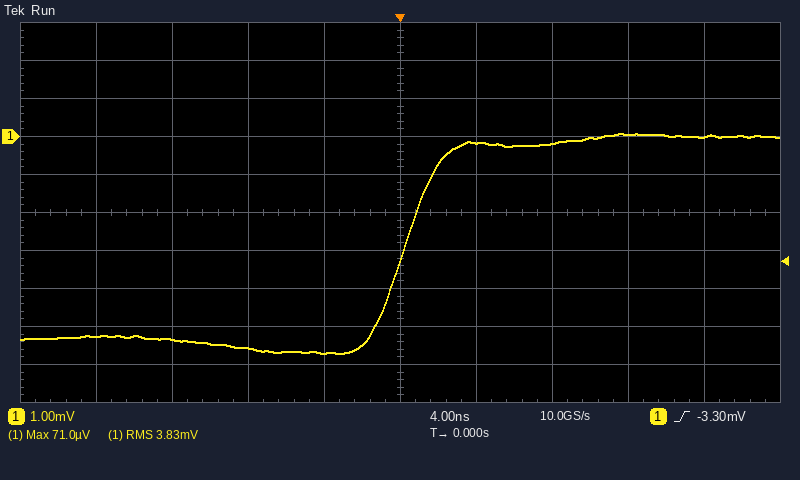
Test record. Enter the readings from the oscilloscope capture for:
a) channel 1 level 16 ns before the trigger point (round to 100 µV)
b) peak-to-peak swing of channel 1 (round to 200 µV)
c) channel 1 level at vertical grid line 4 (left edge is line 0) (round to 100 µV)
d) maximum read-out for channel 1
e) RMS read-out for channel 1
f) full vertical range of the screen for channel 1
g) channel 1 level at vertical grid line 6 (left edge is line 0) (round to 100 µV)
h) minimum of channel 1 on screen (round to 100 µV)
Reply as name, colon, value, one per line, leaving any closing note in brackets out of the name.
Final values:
channel 1 level 16 ns before the trigger point: -5.3 mV
peak-to-peak swing of channel 1: 5.8 mV
channel 1 level at vertical grid line 4 (left edge is line 0): -5.7 mV
maximum read-out for channel 1: 71.0 µV
RMS read-out for channel 1: 3.83 mV
full vertical range of the screen for channel 1: 10 mV
channel 1 level at vertical grid line 6 (left edge is line 0): -200 µV
minimum of channel 1 on screen: -5.7 mV
